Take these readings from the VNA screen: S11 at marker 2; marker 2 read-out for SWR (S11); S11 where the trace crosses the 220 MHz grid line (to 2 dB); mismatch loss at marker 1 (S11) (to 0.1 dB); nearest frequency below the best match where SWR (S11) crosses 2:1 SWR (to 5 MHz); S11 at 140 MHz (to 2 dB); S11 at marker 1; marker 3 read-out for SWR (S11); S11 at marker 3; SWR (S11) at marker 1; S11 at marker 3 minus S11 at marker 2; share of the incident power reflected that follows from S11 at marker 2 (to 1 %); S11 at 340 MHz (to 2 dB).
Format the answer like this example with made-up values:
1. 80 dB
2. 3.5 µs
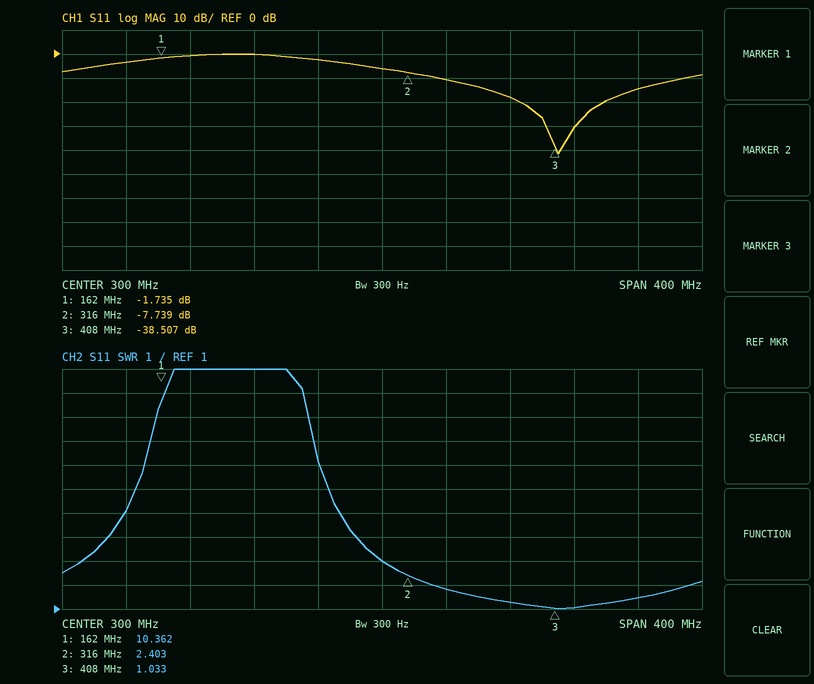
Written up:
1. -7.739 dB
2. 2.403
3. 0 dB
4. 4.8 dB
5. 330 MHz
6. -4 dB
7. -1.735 dB
8. 1.033
9. -38.507 dB
10. 10.362
11. -30.768 dB
12. 17 %
13. -10 dB
